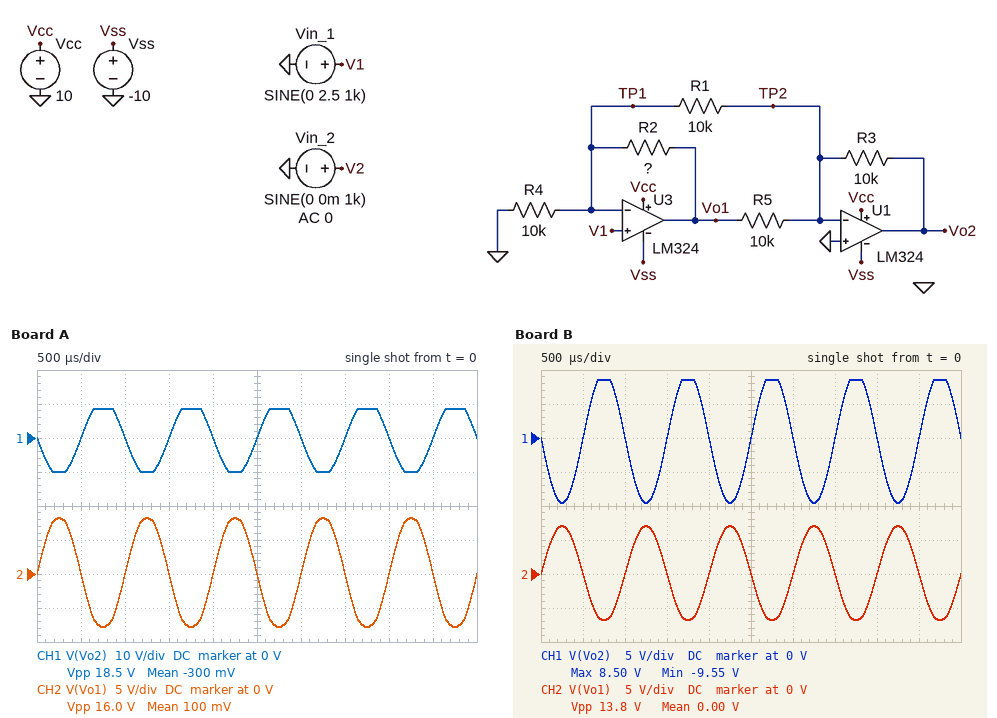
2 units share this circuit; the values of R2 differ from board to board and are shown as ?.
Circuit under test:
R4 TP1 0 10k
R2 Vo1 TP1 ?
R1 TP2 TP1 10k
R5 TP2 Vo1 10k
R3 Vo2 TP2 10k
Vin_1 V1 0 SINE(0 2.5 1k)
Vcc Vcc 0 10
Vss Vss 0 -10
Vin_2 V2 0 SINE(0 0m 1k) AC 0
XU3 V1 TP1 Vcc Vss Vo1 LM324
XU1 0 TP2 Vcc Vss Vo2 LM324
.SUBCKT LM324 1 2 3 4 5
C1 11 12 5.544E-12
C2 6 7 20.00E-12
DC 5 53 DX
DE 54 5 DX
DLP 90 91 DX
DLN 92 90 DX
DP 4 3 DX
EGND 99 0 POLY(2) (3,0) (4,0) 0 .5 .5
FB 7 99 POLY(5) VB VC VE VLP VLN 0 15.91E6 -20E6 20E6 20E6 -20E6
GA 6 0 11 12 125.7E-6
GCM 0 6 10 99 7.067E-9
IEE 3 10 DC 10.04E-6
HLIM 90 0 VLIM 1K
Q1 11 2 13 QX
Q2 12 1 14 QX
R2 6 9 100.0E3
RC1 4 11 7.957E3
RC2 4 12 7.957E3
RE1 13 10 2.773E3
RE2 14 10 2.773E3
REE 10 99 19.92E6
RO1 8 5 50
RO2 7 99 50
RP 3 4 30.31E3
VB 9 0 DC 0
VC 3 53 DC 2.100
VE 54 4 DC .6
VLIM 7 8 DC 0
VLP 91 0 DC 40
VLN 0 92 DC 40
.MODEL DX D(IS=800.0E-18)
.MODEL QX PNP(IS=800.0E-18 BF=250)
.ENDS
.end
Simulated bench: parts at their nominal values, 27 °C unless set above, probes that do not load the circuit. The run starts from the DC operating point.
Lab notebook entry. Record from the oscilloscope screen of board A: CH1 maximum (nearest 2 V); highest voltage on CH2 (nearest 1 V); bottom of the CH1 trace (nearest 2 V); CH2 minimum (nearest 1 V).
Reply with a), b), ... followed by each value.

a) 8 V
b) 8 V
c) -10 V
d) -8 V
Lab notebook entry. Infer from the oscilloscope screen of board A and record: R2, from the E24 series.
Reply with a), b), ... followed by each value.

a) 12 kΩ
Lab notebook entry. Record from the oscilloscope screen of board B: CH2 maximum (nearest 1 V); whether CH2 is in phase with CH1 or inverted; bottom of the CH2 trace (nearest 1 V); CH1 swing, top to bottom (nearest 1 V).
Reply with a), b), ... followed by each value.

a) 7 V
b) inverted
c) -7 V
d) 18 V
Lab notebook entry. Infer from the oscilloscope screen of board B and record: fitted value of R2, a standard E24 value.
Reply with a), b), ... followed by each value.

a) 9.1 kΩ
